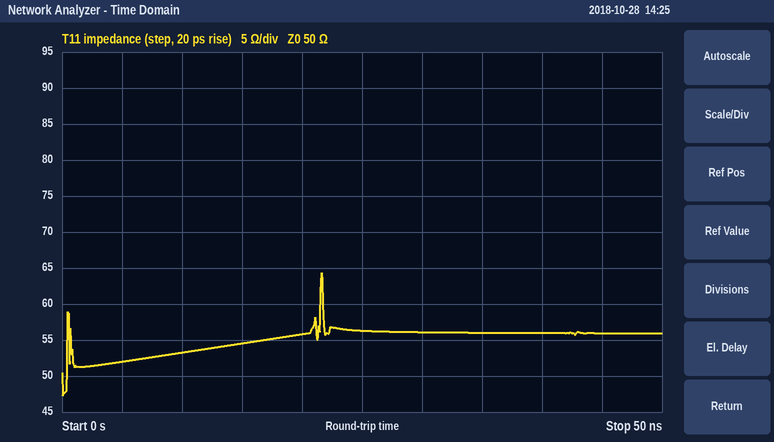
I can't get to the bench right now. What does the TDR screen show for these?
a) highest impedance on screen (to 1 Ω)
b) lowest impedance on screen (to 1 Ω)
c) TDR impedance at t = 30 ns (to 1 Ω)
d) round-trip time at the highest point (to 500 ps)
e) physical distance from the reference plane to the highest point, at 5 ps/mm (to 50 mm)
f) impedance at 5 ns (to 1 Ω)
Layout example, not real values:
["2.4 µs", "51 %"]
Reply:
["64 Ω", "47 Ω", "56 Ω", "21.5 ns", "2.15 m", "52 Ω"]
